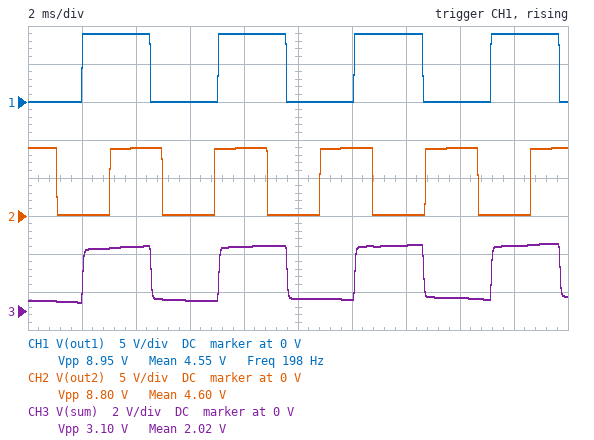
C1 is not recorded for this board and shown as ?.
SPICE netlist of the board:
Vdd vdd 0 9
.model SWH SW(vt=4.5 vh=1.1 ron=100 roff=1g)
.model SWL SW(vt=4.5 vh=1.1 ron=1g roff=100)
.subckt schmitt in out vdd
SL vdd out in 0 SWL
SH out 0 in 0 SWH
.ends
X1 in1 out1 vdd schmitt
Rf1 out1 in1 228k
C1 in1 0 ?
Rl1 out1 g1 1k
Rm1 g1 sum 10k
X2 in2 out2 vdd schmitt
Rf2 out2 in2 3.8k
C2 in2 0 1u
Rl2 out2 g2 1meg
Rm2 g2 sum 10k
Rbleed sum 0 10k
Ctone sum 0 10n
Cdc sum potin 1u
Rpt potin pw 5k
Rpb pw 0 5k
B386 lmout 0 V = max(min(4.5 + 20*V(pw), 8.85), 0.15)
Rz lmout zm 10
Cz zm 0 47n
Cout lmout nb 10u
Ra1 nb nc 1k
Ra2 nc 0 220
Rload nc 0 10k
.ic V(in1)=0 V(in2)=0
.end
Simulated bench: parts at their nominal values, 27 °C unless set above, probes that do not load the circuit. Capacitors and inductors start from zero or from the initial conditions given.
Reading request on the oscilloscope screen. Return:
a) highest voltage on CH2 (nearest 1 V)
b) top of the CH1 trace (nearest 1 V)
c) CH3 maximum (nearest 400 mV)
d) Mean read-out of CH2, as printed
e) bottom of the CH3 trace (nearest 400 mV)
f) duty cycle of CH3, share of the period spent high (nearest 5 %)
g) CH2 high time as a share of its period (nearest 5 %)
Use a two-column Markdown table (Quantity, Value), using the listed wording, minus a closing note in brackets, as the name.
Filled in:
| Quantity | Value |
|---|---|
| highest voltage on CH2 | 9 V |
| top of the CH1 trace | 9 V |
| CH3 maximum | 3.6 V |
| Mean read-out of CH2, as printed | 4.60 V |
| bottom of the CH3 trace | 400 mV |
| duty cycle of CH3, share of the period spent high | 50 % |
| CH2 high time as a share of its period | 50 % |
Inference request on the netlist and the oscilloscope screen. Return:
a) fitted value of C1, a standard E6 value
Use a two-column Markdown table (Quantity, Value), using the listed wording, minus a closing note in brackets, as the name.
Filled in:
| Quantity | Value |
|---|---|
| fitted value of C1, a standard E6 value | 22 nF |
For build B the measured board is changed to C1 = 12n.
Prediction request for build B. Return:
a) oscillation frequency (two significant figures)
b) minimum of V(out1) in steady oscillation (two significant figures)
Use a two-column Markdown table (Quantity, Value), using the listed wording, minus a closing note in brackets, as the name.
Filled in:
| Quantity | Value |
|---|---|
| oscillation frequency | 360 Hz |
| minimum of V(out1) in steady oscillation | 5.3 mV |
